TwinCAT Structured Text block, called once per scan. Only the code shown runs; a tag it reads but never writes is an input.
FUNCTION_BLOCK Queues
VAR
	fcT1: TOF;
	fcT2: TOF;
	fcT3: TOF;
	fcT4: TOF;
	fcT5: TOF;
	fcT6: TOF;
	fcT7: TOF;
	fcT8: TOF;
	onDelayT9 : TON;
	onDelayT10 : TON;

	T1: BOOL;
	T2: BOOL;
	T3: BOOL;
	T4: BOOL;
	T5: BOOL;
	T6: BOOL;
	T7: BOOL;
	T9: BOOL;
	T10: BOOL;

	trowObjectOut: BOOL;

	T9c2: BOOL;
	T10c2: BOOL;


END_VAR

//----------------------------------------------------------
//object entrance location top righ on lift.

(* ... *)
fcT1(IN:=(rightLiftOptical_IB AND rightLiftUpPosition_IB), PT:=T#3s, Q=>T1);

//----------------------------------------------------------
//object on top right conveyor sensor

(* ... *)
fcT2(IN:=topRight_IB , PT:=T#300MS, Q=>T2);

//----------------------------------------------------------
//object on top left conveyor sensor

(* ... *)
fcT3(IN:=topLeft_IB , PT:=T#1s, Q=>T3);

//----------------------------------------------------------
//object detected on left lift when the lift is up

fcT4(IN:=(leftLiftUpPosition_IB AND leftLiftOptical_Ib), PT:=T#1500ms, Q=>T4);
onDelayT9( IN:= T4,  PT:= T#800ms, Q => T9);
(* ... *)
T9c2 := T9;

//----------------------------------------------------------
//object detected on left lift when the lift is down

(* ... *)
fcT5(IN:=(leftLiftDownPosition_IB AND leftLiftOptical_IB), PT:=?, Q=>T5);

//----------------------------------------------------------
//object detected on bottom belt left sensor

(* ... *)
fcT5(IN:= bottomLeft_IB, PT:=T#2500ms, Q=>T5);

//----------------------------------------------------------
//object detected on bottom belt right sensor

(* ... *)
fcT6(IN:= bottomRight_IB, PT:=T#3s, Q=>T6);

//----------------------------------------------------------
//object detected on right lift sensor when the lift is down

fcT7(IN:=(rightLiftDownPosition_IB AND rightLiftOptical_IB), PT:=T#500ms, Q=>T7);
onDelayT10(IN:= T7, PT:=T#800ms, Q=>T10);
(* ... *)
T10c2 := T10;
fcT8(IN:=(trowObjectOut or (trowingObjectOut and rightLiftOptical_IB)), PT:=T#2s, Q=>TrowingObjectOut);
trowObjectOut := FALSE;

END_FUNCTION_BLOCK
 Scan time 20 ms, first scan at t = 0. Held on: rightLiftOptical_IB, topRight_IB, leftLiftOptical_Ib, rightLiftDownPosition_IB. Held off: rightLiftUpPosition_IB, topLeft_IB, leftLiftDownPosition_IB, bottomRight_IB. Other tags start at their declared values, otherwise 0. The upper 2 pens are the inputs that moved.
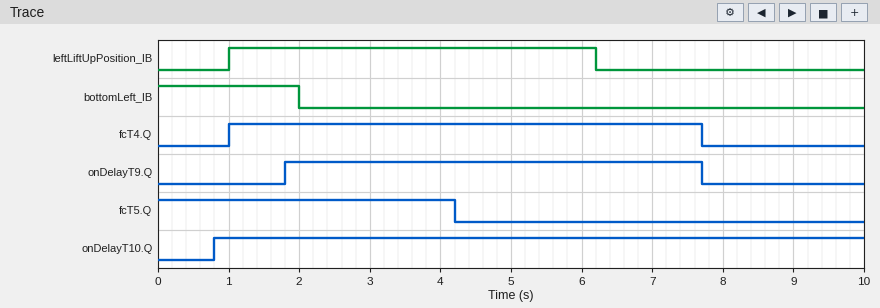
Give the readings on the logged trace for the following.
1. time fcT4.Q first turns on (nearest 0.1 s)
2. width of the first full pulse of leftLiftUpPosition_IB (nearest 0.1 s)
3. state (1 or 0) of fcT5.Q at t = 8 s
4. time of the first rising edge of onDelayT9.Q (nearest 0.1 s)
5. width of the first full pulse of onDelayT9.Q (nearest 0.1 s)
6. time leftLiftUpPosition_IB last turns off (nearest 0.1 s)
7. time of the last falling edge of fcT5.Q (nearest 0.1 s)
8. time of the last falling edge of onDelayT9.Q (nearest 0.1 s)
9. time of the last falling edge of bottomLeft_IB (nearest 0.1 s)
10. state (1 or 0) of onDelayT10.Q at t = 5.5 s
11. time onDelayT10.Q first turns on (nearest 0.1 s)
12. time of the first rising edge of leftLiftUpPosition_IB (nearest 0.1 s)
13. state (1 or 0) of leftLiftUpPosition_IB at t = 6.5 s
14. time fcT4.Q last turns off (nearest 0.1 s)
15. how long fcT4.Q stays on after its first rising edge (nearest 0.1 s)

1.0 s
5.2 s
0
1.8 s
5.9 s
6.2 s
4.2 s
7.7 s
2.0 s
1
0.8 s
1.0 s
0
7.7 s
6.7 s
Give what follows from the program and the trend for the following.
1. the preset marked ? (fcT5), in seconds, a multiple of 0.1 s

2.2 s
